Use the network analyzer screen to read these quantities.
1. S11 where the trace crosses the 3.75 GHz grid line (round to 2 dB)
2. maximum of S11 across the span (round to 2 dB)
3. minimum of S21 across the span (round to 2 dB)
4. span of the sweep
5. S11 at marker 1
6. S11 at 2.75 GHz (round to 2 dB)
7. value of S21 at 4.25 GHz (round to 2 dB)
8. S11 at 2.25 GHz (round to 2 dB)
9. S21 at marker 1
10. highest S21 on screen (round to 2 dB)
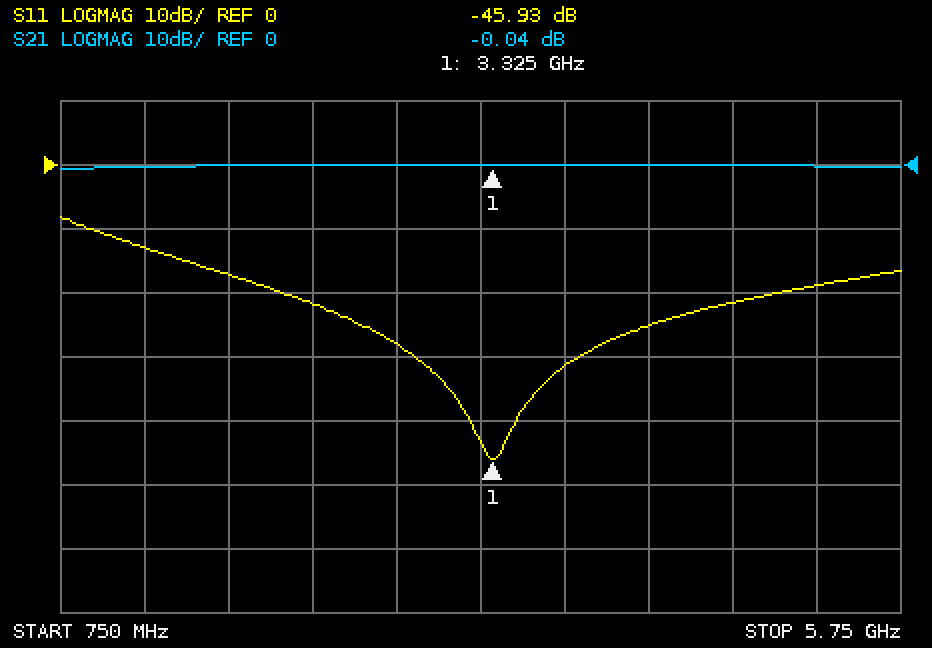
-32 dB
-8 dB
0 dB
5 GHz
-45.93 dB
-28 dB
0 dB
-22 dB
-0.04 dB
0 dB
